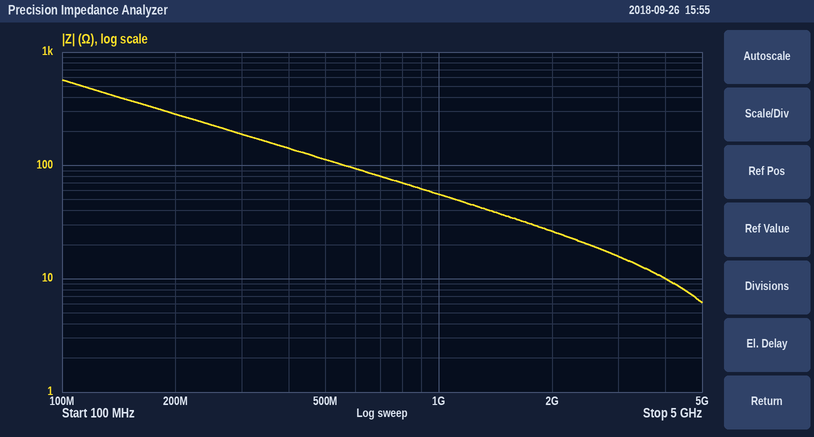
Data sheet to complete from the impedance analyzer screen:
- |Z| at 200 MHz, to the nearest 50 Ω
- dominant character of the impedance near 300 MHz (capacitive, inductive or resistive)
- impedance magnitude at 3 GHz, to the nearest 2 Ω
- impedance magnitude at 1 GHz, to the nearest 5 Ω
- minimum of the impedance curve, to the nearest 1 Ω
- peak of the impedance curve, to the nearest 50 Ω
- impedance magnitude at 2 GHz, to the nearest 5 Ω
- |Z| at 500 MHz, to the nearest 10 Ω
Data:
300 Ω
capacitive
16 Ω
55 Ω
6 Ω
550 Ω
25 Ω
110 Ω
